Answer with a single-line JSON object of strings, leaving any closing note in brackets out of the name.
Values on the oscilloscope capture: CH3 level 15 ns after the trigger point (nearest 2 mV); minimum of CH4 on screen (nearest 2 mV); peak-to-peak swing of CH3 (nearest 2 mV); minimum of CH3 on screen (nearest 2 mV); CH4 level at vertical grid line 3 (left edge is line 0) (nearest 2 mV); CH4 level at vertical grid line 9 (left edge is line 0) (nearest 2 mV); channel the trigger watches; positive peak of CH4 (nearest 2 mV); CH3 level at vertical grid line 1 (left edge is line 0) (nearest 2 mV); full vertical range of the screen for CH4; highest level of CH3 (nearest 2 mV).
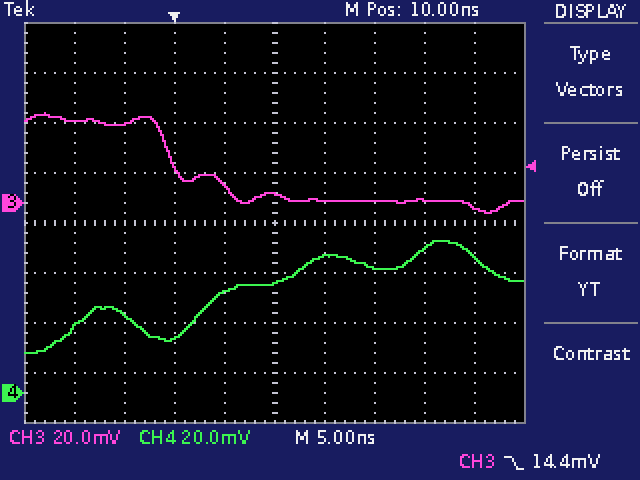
{"CH3 level 15 ns after the trigger point": "0 mV", "minimum of CH4 on screen": "16 mV", "peak-to-peak swing of CH3": "40 mV", "minimum of CH3 on screen": "-4 mV", "CH4 level at vertical grid line 3 (left edge is line 0)": "22 mV", "CH4 level at vertical grid line 9 (left edge is line 0)": "54 mV", "channel the trigger watches": "CH3", "positive peak of CH4": "60 mV", "CH3 level at vertical grid line 1 (left edge is line 0)": "32 mV", "full vertical range of the screen for CH4": "160 mV", "highest level of CH3": "36 mV"}
